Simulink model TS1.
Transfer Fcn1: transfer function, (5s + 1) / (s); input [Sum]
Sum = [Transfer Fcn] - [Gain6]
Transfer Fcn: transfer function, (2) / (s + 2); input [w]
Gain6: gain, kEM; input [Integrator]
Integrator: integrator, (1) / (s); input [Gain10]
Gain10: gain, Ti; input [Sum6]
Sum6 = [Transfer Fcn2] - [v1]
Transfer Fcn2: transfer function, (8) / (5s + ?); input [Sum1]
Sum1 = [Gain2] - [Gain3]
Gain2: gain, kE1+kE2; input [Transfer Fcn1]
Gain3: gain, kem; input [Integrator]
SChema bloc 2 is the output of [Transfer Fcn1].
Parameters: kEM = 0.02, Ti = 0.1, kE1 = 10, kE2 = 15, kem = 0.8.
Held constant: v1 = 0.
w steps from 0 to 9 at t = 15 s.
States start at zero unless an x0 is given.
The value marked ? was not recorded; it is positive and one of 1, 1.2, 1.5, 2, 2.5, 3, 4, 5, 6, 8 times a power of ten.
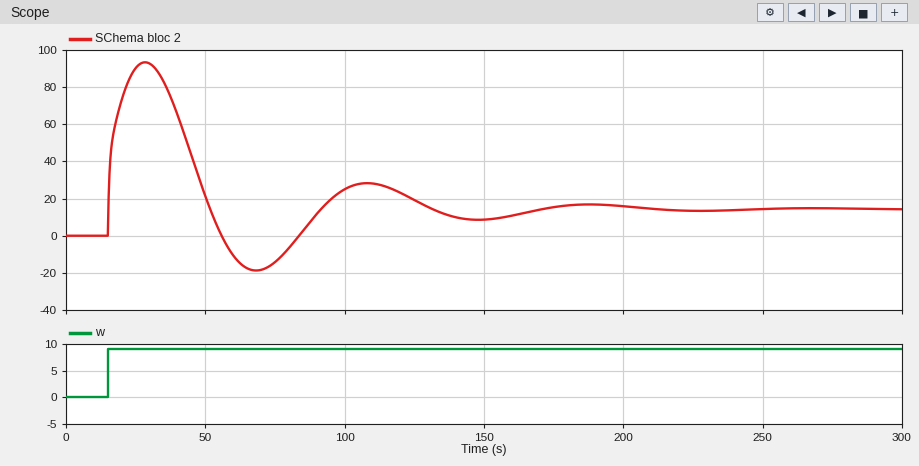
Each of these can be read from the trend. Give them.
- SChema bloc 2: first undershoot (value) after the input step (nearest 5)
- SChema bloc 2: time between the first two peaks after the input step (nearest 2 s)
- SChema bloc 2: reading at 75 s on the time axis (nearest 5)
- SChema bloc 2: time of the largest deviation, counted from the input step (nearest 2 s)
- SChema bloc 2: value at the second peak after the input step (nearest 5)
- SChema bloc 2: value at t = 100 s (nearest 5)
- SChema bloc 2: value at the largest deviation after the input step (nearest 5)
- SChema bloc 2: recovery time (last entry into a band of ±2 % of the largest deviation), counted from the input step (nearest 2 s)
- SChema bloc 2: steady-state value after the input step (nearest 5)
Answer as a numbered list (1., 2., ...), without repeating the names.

1. -20
2. 80 s
3. -15
4. 14 s
5. 30
6. 25
7. 95
8. 182 s
9. 15
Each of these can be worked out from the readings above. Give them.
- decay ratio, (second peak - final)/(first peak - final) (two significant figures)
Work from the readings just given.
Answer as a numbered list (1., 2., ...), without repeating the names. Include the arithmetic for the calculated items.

1. (30 - 15) / (95 - 15) = 0.19
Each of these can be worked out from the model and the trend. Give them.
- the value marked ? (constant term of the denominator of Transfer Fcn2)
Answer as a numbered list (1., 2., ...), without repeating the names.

1. 60
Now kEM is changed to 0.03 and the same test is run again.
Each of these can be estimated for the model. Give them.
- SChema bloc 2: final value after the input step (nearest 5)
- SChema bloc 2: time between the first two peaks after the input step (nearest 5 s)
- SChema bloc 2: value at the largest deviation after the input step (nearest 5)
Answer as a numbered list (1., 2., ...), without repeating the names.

1. 10
2. 65 s
3. 75
